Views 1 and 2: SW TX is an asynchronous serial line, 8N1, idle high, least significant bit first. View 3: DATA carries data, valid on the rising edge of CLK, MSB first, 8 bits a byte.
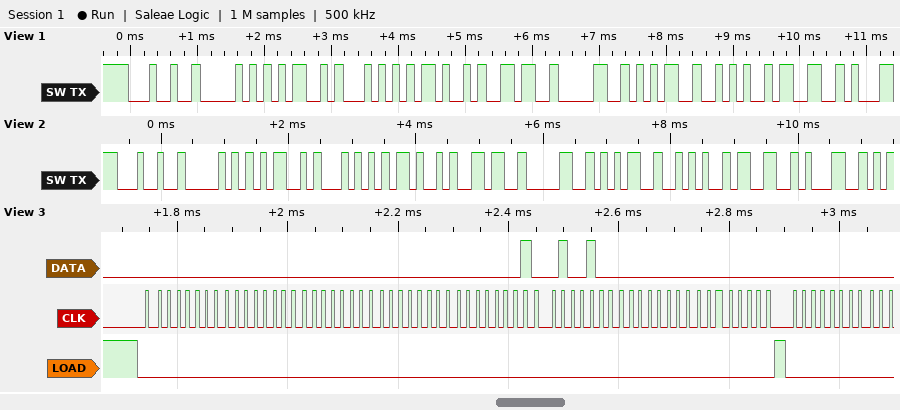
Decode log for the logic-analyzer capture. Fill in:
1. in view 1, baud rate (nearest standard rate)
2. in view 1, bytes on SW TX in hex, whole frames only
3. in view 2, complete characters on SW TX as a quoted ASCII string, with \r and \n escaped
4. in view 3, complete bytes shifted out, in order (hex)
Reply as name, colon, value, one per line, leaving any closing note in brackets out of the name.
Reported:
in view 1, baud rate: 9600 baud
in view 1, bytes on SW TX in hex, whole frames only: 0x24 0x50 0x4D 0x54 0x4B 0x36 0x30 0x35 0x2A 0x33
in view 2, complete characters on SW TX as a quoted ASCII string, with \r and \n escaped: "$PMTK605*31"
in view 3, complete bytes shifted out, in order: 00 00 00 00 01 24 00 00 00
